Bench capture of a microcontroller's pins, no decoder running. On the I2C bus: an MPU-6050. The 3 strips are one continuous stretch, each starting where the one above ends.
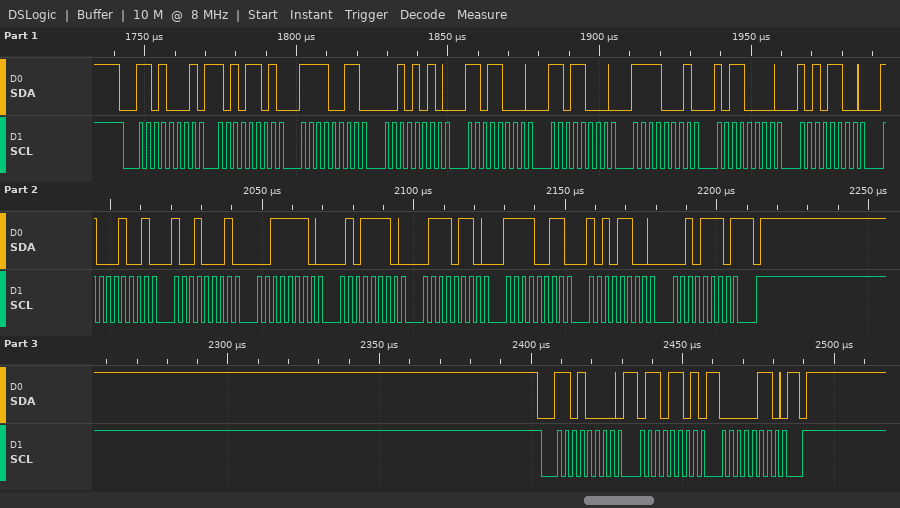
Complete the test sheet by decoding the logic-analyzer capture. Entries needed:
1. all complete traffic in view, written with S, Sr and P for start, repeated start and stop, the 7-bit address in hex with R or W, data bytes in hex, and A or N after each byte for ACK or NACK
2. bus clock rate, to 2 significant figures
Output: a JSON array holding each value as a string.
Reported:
["S 68R A AD A F3 A 2A A D8 A D8 A F1 A B0 A AC A 89 A 91 A 3E A 5E A 76 A F3 A AC A 2E N P S 68W A 6D A 06 A P", "400 kHz"]
